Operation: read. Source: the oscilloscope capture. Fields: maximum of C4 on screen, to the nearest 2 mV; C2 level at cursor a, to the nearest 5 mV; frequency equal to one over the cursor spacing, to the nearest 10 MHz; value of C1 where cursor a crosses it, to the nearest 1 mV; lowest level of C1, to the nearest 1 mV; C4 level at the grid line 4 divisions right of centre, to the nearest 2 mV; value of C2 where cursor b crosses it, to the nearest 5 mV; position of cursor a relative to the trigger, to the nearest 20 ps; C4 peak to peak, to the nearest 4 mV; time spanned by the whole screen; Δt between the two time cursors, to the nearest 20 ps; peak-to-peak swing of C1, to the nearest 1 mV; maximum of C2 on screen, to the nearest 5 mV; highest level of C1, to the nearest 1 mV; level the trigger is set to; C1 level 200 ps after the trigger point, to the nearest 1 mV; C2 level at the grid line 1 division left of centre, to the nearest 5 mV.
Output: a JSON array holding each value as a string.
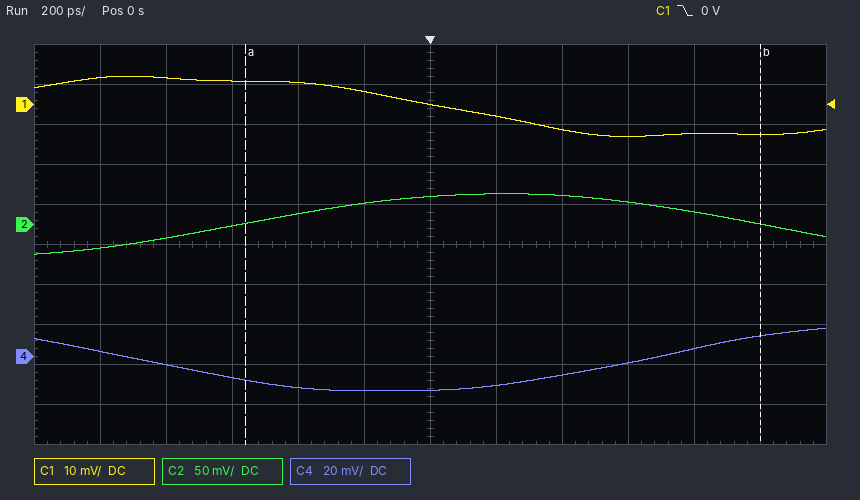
["14 mV", "0 mV", "640 MHz", "6 mV", "-8 mV", "4 mV", "0 mV", "-560 ps", "32 mV", "2.4 ns", "1.56 ns", "15 mV", "40 mV", "7 mV", "0 V", "-3 mV", "25 mV"]
